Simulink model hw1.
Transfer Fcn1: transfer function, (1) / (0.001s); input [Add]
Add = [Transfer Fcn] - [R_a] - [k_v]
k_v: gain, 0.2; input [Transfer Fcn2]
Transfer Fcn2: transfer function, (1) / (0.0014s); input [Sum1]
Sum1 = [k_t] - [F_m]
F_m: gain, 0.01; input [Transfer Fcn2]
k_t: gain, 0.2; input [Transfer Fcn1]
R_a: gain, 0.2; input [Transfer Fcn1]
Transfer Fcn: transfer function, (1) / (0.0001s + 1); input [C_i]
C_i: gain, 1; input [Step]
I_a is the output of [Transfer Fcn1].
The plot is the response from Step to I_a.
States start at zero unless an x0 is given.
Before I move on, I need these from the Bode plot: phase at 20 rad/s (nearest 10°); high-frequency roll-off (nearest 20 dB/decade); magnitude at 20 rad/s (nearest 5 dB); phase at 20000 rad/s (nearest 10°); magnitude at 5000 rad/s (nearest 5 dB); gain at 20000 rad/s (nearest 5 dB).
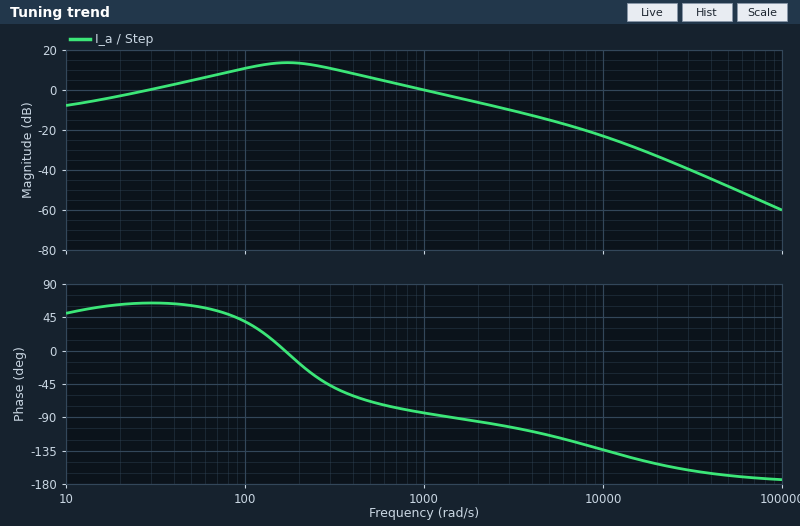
60°
-40 dB/decade
-5 dB
-150°
-15 dB
-35 dB
